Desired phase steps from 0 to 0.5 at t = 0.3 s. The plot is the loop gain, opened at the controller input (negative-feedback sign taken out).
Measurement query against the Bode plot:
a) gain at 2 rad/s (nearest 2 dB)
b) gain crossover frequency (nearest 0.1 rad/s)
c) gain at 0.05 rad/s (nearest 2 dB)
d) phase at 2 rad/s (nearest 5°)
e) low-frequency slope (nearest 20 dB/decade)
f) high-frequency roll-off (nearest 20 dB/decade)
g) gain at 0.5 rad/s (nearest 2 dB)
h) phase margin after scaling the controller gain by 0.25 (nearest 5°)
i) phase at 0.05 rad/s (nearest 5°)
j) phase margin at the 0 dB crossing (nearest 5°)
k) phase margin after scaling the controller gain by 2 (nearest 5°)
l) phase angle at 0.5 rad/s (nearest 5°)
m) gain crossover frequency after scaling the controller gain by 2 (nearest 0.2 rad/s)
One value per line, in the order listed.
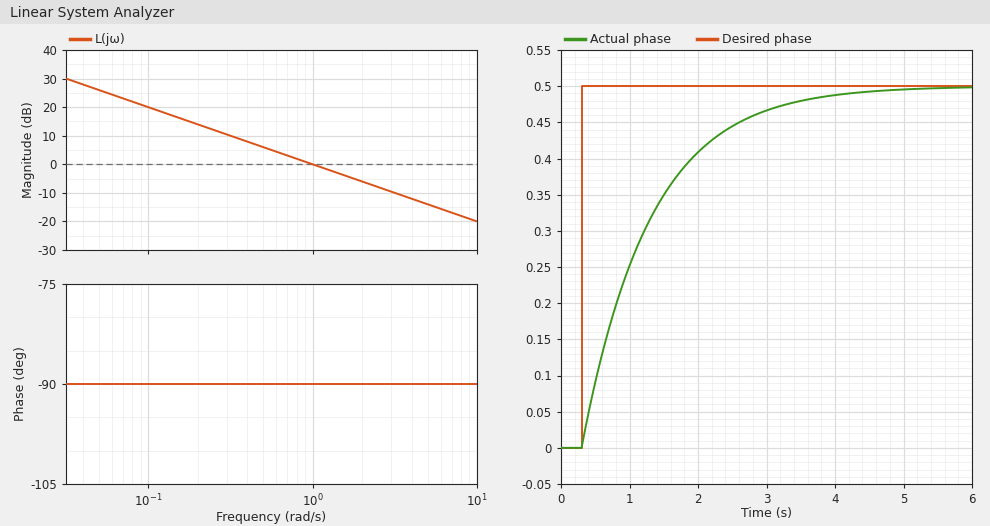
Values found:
-6 dB
1.0 rad/s
26 dB
-90°
-20 dB/decade
-20 dB/decade
6 dB
90°
-90°
90°
90°
-90°
2.0 rad/s
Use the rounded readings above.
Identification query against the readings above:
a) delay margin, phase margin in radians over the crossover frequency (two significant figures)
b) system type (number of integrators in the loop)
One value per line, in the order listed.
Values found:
1.6 s
1
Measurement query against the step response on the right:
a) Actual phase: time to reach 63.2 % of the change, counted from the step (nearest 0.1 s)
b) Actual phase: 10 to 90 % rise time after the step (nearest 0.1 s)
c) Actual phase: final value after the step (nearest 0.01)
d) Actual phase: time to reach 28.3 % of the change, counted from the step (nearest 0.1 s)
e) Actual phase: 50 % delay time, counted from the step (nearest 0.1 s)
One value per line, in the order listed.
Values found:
1.0 s
2.2 s
0.50
0.3 s
0.7 s
